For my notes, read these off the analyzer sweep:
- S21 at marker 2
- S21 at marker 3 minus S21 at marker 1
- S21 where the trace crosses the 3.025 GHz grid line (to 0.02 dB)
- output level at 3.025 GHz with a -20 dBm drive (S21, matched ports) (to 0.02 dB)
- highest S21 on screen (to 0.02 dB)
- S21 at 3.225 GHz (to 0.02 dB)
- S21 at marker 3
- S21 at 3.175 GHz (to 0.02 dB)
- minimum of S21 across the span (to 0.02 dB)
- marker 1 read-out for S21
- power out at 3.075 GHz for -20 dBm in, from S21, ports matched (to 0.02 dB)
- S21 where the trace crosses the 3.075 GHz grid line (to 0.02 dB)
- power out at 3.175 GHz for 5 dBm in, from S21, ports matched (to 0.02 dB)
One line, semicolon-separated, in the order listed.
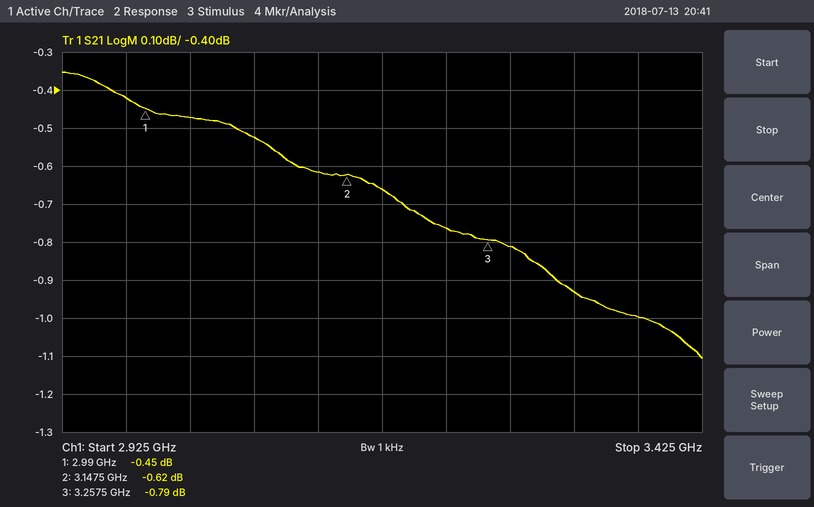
-0.62 dB; -0.34 dB; -0.48 dB; -20.48 dBm; -0.36 dB; -0.76 dB; -0.79 dB; -0.66 dB; -1.10 dB; -0.45 dB; -20.52 dBm; -0.52 dB; 4.34 dBm
